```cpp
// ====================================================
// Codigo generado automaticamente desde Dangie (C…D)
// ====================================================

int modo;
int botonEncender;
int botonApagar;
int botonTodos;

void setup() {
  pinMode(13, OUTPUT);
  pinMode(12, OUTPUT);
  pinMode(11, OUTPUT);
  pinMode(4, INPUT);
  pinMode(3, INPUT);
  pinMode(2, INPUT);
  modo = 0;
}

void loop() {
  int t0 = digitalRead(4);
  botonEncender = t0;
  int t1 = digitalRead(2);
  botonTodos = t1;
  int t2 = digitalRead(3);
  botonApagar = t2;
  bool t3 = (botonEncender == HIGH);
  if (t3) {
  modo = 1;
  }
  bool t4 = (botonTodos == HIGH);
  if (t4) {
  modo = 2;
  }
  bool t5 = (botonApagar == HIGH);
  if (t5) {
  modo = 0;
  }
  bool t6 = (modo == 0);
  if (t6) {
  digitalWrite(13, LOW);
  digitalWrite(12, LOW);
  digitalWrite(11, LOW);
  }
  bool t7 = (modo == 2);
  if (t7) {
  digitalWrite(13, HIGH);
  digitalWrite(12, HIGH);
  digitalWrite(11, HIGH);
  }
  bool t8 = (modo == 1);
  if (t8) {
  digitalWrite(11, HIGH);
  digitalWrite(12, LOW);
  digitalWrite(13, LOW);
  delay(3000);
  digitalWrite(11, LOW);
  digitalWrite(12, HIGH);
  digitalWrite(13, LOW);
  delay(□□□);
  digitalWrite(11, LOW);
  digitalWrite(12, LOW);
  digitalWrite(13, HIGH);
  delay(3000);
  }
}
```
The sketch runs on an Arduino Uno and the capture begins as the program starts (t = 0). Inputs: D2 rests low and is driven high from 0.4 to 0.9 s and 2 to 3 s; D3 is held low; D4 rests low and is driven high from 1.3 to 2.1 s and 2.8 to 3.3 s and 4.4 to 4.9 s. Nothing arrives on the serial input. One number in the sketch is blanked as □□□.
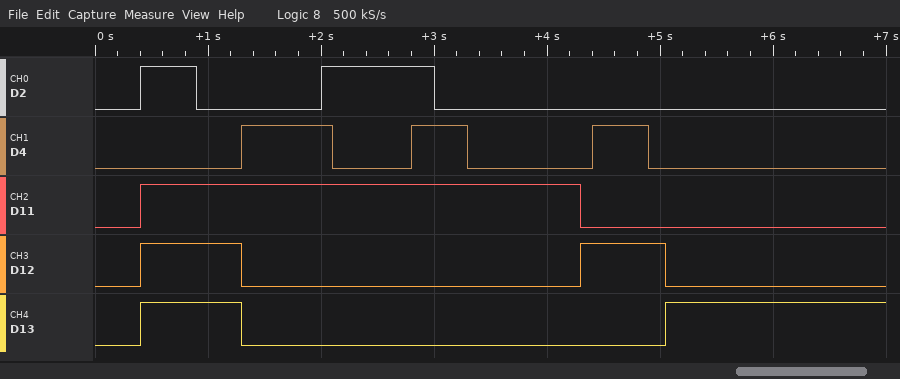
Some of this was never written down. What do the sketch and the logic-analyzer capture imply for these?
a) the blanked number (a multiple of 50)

750
